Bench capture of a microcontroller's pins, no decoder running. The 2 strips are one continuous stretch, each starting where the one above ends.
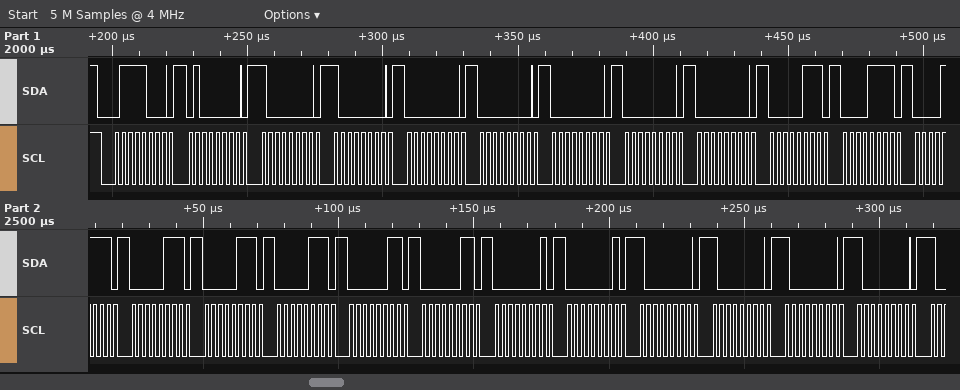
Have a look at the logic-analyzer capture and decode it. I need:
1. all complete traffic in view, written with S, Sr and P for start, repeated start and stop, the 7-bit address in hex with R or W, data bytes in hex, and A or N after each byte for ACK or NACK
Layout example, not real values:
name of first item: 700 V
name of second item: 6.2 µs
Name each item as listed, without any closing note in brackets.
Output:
all complete traffic in view, written with S, Sr and P for start, repeated start and stop, the 7-bit address in hex with R or W, data bytes in hex, and A or N after each byte for ACK or NACK: S 3CW A 40 A 80 A 80 A 00 A 00 A 00 A 00 A 00 A 07 A 0F A 0F A 07 A 07 A 07 A 03 A 03 A 01 A 01 A 80 A 80 A 80 A 80 A
